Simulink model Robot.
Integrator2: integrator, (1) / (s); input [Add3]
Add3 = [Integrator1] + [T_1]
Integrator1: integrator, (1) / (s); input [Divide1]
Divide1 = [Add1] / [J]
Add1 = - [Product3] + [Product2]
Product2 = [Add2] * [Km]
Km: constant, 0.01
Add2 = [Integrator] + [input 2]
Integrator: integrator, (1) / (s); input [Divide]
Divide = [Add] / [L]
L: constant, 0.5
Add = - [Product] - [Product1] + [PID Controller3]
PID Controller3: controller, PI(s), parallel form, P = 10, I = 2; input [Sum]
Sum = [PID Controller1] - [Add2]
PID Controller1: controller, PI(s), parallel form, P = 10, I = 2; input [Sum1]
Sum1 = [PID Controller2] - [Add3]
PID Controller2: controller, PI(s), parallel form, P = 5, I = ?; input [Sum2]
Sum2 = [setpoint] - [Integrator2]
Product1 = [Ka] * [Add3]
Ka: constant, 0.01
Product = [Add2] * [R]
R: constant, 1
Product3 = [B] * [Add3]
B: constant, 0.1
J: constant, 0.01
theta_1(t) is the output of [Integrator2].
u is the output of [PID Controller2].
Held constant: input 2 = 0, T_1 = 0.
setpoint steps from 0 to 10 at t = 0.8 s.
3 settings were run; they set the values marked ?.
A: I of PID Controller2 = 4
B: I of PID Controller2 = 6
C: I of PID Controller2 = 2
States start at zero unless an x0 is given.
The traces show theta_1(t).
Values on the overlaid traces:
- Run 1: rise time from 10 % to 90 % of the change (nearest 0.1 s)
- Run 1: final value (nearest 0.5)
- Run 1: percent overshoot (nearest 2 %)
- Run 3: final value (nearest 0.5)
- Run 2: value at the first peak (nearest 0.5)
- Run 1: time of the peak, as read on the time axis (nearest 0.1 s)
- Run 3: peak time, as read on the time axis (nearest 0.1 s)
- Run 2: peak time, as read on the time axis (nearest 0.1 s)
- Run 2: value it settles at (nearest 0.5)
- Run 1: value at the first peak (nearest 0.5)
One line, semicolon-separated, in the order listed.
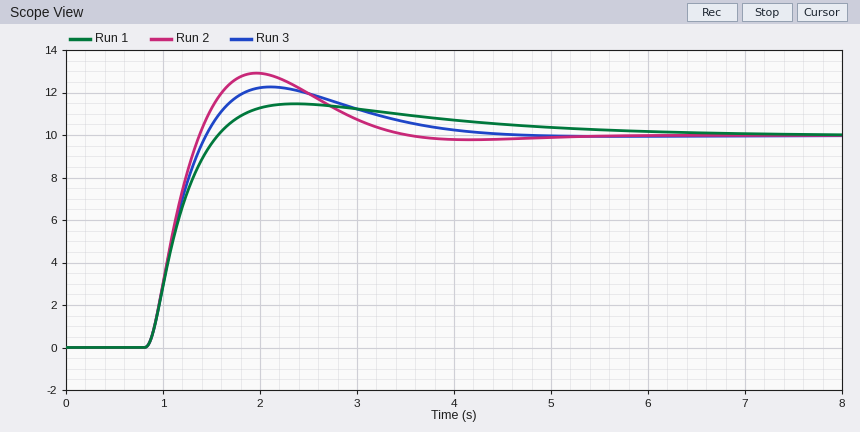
0.5 s; 10.0; 14 %; 10.0; 13.0; 2.4 s; 2.1 s; 2.0 s; 10.0; 11.5
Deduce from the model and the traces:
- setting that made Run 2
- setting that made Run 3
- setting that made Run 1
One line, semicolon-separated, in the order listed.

B; A; C
